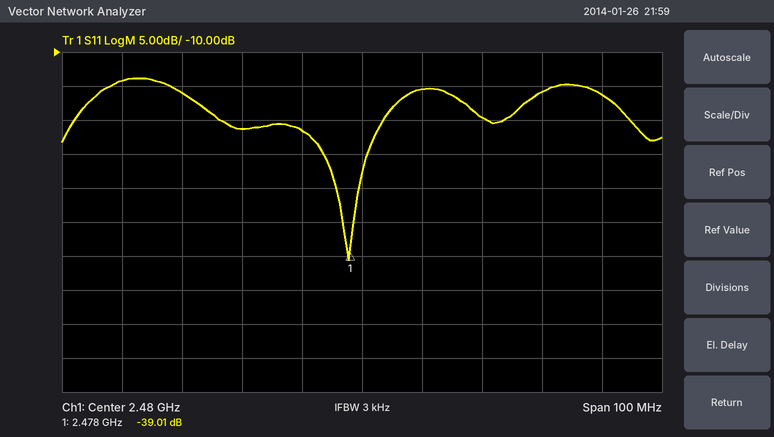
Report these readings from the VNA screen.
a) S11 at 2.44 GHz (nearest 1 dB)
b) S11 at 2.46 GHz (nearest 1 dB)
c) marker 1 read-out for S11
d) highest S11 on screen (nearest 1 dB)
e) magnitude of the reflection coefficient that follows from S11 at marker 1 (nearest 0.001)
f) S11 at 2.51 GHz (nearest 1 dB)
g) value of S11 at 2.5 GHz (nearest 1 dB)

-14 dB
-21 dB
-39.01 dB
-14 dB
0.011
-16 dB
-20 dB
